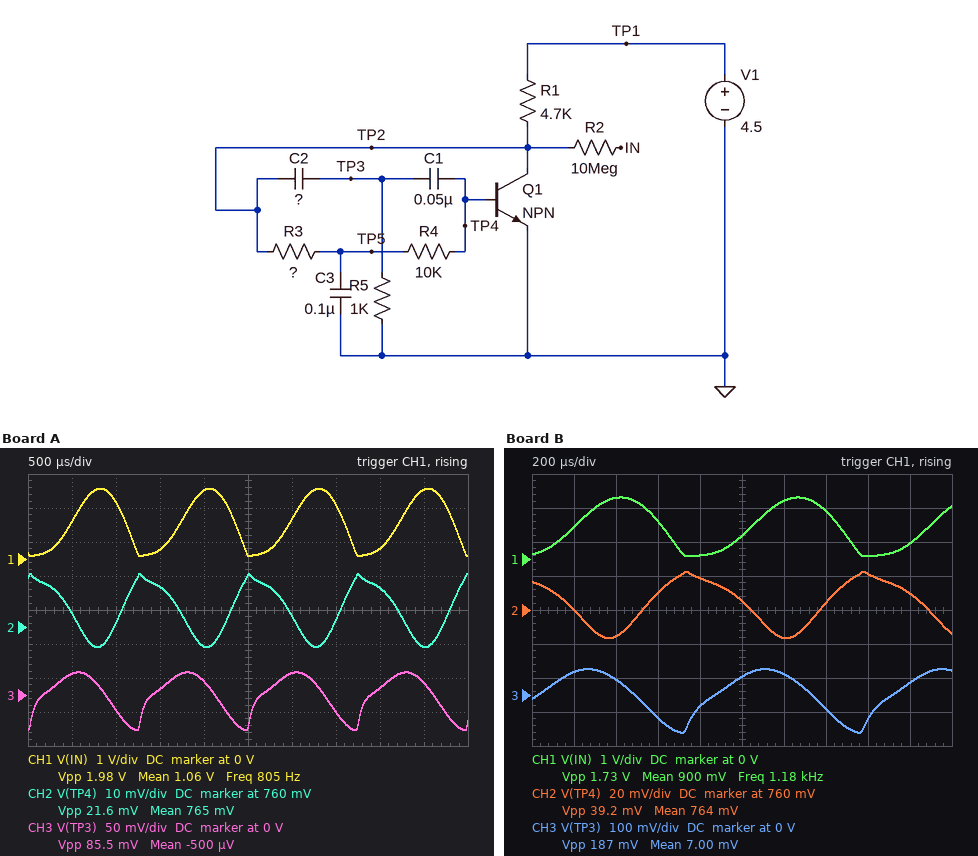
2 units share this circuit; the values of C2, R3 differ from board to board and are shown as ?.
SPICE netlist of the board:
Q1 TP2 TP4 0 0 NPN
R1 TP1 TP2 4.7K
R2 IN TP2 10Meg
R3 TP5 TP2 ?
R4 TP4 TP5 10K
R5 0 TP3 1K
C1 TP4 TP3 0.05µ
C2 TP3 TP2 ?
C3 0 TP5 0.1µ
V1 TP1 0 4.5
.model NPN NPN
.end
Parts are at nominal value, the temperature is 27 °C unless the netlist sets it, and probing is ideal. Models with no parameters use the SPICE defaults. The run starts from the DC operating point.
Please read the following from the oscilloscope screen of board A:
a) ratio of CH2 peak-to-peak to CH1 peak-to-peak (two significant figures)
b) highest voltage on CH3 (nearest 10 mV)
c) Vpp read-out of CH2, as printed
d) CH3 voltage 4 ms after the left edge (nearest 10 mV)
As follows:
0.011
30 mV
21.6 mV
10 mV
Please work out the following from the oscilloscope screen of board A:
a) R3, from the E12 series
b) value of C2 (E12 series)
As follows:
22 kΩ
8.2 nF
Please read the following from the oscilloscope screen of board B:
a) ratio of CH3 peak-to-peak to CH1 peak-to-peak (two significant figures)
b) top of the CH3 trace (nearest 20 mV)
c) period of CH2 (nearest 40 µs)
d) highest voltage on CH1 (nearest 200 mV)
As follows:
0.11
80 mV
840 µs
1.8 V
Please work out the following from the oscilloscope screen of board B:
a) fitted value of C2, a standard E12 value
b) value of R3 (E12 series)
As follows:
15 nF
3.3 kΩ
